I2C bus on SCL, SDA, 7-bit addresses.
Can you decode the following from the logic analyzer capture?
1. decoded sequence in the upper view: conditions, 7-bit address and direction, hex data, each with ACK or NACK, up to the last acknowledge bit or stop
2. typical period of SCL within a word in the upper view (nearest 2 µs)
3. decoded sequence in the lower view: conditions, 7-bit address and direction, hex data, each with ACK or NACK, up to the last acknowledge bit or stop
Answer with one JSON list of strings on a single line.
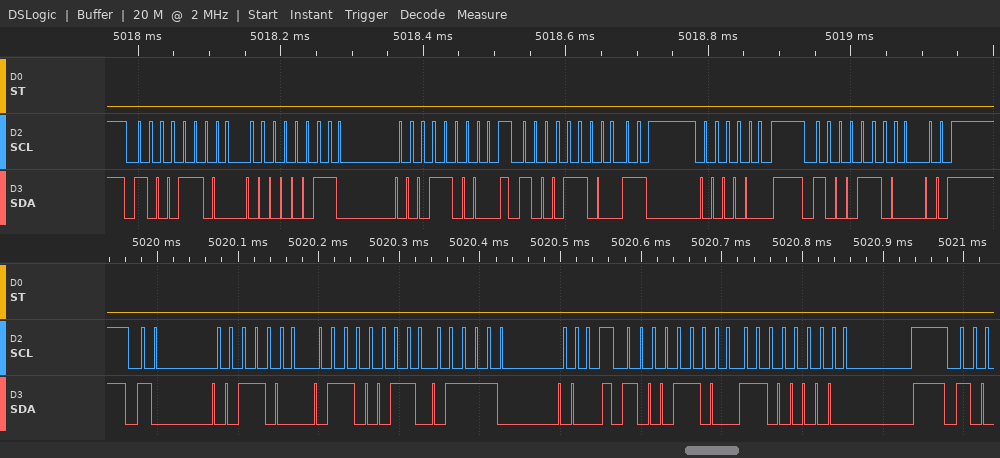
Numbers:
["start, address 46 write ACK, 03 ACK, 18 ACK, stop, start, address 46 write ACK, C0 ACK, stop, start, address 46 write ACK", "16 µs", "start, address 46 write ACK, 63 ACK, 78 ACK, stop, start, address 46 write ACK, C0 ACK, stop"]
